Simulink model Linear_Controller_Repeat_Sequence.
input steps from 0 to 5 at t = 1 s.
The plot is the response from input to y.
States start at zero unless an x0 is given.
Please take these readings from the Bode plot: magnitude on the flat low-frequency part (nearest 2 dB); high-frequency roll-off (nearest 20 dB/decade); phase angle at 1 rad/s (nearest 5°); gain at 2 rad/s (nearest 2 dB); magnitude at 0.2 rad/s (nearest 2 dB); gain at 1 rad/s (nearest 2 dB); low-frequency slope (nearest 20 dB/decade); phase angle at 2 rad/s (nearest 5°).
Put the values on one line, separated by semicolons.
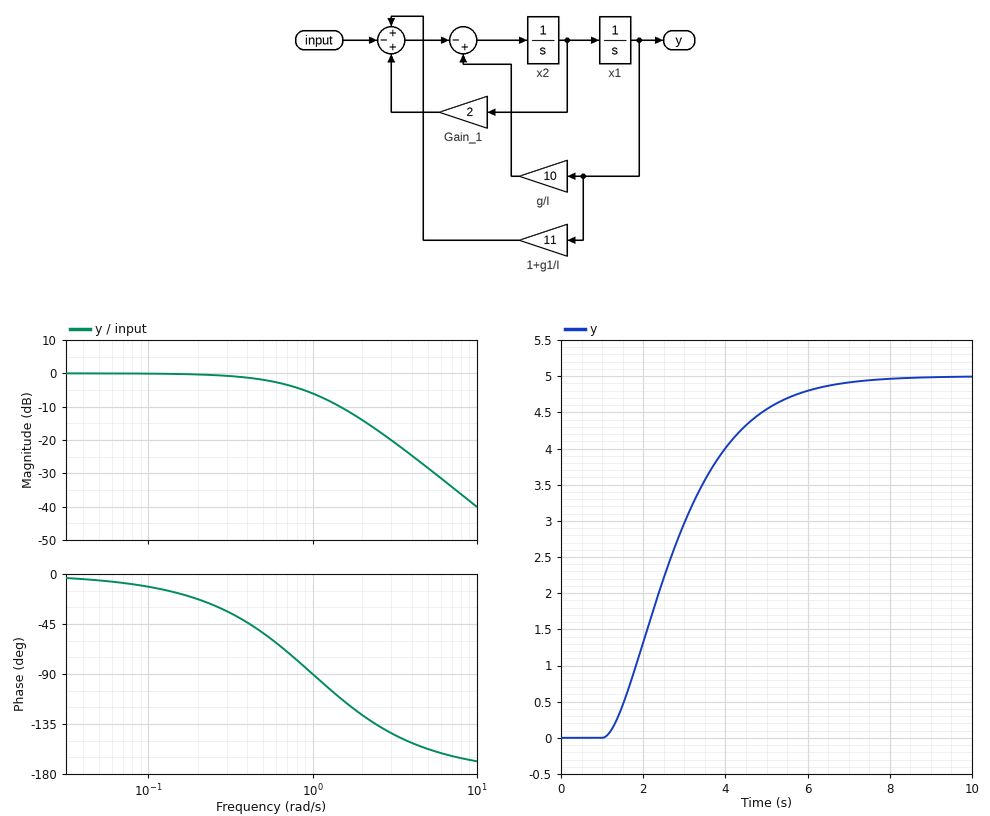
0 dB; -40 dB/decade; -90°; -14 dB; 0 dB; -6 dB; 0 dB/decade; -125°
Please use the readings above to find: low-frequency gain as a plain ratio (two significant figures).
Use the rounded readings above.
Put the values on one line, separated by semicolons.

1.0
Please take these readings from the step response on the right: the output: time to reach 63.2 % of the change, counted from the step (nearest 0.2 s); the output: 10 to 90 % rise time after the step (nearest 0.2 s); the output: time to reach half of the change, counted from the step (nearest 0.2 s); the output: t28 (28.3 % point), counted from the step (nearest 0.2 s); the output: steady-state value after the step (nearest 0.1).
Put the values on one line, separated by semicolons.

2.2 s; 3.4 s; 1.6 s; 1.0 s; 5.0
